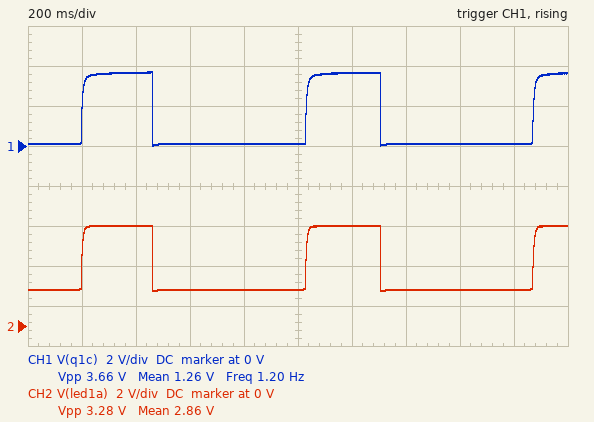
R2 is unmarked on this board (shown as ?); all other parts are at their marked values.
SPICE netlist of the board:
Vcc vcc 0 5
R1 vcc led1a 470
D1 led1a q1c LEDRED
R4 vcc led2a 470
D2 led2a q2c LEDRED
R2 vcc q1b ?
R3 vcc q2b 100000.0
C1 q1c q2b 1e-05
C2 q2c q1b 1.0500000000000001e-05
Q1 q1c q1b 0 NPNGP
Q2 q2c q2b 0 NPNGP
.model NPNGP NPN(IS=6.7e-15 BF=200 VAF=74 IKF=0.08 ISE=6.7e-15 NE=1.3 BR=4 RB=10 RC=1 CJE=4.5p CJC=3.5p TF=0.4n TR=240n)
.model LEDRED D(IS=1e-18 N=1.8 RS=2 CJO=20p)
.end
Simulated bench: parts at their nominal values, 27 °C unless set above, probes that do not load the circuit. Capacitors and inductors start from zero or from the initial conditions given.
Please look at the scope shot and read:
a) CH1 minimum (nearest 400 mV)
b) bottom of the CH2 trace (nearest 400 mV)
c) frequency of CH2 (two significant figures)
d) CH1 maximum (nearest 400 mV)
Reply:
0 V
1.6 V
1.2 Hz
3.6 V
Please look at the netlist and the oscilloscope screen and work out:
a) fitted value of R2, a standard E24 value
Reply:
51 kΩ
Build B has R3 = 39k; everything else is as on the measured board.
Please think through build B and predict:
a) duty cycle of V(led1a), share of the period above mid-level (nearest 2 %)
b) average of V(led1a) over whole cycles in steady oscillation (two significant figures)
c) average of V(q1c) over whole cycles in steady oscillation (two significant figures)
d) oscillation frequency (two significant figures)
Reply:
58 %
3.6 V
2.1 V
1.9 Hz
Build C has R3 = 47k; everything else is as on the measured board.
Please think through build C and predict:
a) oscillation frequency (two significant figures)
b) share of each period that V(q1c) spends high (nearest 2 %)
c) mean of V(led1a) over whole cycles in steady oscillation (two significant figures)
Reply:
1.8 Hz
52 %
3.5 V
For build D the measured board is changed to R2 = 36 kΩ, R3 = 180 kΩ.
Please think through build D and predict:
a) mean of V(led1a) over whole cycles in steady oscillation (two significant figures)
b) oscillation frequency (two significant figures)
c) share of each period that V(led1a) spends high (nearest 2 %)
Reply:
2.1 V
870 mHz
10 %
